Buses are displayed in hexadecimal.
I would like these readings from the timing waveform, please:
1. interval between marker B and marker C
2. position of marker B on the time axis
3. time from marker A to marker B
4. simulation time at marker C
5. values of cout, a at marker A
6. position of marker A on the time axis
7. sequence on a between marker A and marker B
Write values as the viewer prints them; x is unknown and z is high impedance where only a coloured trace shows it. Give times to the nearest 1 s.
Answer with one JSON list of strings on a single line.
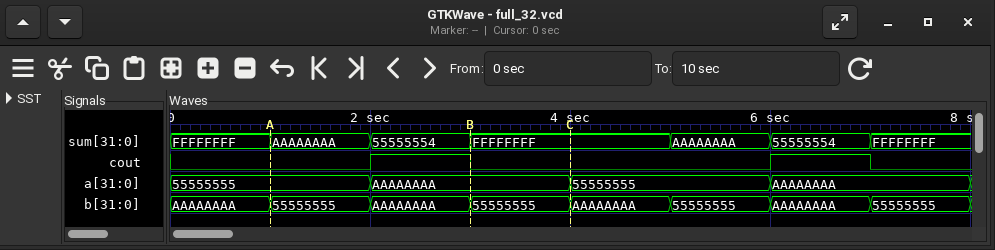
["1 s", "3 s", "2 s", "4 s", "cout=0, a=55555555", "1 s", "55555555, AAAAAAAA"]
